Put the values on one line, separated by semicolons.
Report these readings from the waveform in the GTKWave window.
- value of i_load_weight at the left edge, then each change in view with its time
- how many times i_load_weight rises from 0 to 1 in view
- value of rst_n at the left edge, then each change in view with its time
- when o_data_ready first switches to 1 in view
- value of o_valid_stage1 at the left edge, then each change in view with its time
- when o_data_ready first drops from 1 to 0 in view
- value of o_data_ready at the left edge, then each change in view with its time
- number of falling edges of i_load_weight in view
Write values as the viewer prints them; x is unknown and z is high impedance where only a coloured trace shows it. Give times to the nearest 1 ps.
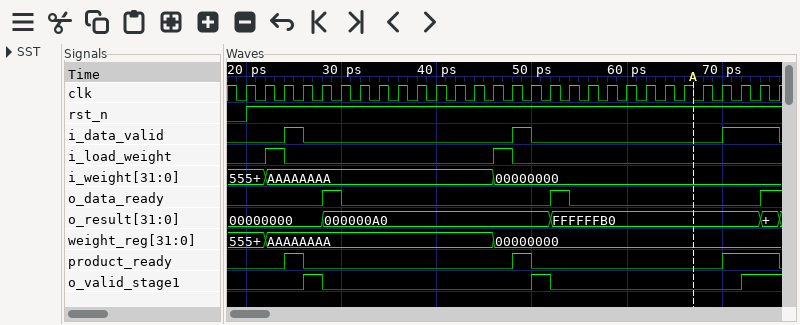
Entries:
0, 1 at 22 ps, 0 at 24 ps, 1 at 46 ps, 0 at 48 ps; 2; 0, 1 at 20 ps; 28 ps; 0, 1 at 26 ps, 0 at 28 ps, 1 at 50 ps, 0 at 52 ps, 1 at 72 ps; 30 ps; 0, 1 at 28 ps, 0 at 30 ps, 1 at 52 ps, 0 at 54 ps, 1 at 74 ps; 2
